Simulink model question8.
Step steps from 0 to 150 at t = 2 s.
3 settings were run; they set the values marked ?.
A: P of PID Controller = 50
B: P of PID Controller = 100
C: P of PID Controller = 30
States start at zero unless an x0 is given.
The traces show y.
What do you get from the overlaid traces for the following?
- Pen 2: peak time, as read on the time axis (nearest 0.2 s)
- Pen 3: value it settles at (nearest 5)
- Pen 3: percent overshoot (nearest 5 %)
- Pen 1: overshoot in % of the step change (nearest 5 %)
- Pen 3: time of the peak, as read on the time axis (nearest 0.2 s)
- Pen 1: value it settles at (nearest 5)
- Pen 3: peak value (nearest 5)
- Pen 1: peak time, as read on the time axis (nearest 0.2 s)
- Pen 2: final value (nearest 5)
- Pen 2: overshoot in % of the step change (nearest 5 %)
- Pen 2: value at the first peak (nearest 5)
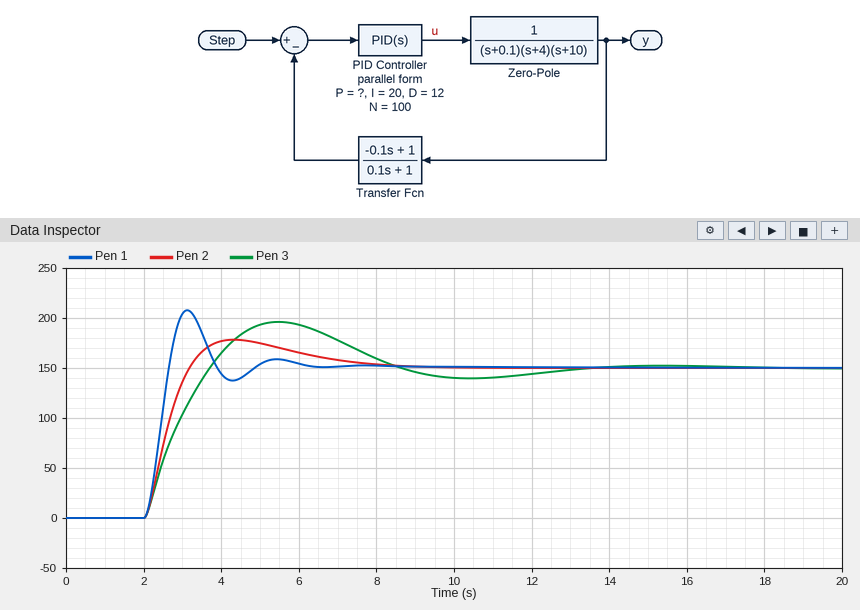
4.4 s
150
30 %
40 %
5.4 s
150
195
3.2 s
150
20 %
180
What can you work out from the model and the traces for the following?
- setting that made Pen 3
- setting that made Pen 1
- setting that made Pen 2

C
B
A
